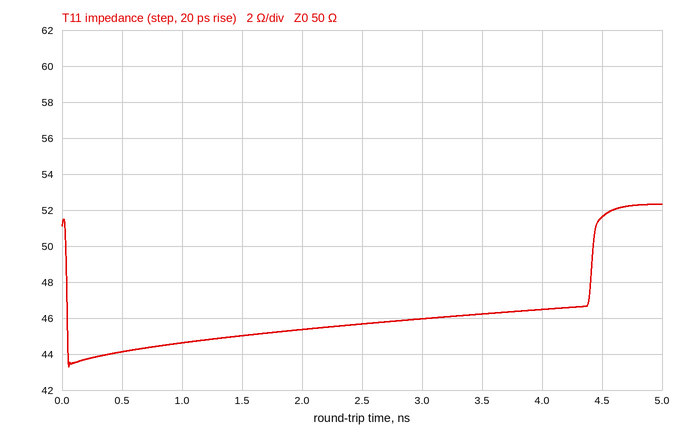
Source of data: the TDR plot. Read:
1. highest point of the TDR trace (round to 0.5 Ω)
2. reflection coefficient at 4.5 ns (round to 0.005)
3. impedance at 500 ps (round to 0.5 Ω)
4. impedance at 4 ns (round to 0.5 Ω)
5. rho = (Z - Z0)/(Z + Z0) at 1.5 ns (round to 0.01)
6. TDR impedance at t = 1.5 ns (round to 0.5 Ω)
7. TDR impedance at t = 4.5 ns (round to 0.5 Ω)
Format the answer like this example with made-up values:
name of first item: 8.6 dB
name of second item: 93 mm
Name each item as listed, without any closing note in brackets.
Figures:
highest point of the TDR trace: 52.5 Ω
reflection coefficient at 4.5 ns: +0.015
impedance at 500 ps: 44.0 Ω
impedance at 4 ns: 46.5 Ω
rho = (Z - Z0)/(Z + Z0) at 1.5 ns: -0.05
TDR impedance at t = 1.5 ns: 45.0 Ω
TDR impedance at t = 4.5 ns: 51.5 Ω
